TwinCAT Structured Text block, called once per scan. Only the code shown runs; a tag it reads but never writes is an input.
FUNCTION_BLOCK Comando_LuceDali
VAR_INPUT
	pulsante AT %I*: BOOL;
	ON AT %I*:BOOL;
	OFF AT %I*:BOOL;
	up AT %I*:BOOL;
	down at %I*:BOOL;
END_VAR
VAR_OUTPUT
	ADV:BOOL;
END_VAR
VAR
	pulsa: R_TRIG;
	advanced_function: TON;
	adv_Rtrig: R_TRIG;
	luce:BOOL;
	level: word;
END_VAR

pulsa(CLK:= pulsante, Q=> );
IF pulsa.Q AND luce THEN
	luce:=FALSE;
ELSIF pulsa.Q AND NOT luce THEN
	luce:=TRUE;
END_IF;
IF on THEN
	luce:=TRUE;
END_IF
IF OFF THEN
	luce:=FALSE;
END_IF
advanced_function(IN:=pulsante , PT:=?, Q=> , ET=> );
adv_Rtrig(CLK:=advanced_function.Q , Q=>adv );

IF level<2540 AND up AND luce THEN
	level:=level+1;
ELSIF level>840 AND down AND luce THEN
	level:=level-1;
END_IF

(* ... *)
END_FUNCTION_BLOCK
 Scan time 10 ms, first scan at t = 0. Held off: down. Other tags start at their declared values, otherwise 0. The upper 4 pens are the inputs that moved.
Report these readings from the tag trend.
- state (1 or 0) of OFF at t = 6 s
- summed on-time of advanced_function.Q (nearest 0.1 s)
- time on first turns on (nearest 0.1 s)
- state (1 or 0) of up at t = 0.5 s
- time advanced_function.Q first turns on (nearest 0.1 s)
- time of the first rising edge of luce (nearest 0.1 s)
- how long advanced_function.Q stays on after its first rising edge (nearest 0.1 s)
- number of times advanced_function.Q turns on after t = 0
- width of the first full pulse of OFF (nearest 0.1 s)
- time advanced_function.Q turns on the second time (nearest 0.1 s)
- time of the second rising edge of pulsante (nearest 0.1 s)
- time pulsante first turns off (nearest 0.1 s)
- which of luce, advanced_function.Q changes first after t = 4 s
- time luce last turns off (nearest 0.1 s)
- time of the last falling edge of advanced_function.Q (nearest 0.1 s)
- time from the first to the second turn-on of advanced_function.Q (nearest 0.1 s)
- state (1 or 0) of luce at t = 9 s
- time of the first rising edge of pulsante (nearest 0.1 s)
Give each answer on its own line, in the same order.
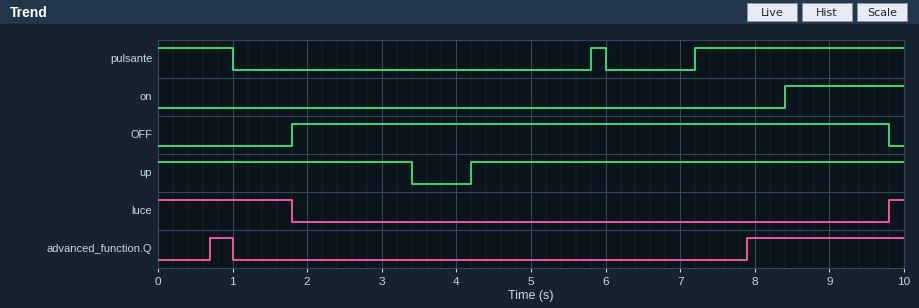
1
2.4 s
8.4 s
1
0.7 s
9.8 s
0.3 s
2
8.0 s
7.9 s
7.2 s
1.0 s
advanced_function.Q
1.8 s
1.0 s
7.2 s
0
5.8 s
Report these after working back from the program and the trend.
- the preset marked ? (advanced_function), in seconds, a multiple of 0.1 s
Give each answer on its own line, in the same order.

0.7 s
